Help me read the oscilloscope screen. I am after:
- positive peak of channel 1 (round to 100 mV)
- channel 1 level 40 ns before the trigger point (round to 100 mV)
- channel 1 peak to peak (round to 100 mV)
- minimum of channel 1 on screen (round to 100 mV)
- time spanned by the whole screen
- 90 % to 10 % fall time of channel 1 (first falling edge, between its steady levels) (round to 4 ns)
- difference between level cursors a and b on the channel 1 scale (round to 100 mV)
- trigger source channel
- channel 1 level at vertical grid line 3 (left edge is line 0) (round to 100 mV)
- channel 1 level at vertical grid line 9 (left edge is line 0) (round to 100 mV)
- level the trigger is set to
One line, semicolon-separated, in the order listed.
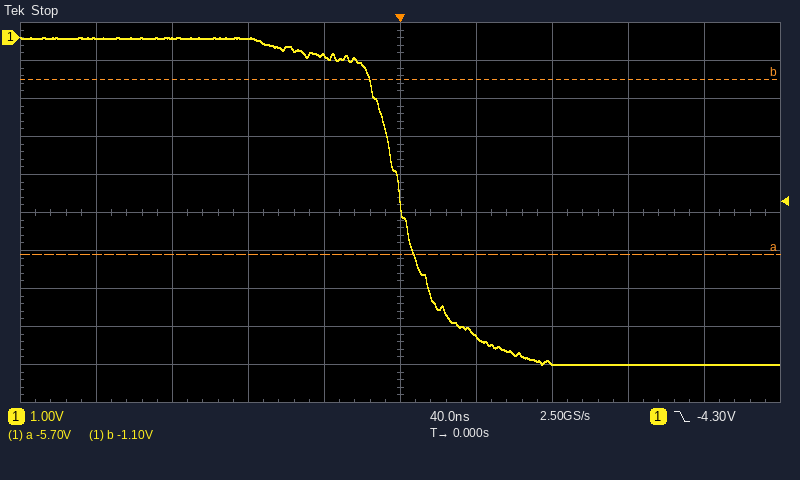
0.0 V; -500 mV; 8.6 V; -8.6 V; 400 ns; 56 ns; 4.6 V; channel 1; 0.0 V; -8.6 V; -4.30 V
